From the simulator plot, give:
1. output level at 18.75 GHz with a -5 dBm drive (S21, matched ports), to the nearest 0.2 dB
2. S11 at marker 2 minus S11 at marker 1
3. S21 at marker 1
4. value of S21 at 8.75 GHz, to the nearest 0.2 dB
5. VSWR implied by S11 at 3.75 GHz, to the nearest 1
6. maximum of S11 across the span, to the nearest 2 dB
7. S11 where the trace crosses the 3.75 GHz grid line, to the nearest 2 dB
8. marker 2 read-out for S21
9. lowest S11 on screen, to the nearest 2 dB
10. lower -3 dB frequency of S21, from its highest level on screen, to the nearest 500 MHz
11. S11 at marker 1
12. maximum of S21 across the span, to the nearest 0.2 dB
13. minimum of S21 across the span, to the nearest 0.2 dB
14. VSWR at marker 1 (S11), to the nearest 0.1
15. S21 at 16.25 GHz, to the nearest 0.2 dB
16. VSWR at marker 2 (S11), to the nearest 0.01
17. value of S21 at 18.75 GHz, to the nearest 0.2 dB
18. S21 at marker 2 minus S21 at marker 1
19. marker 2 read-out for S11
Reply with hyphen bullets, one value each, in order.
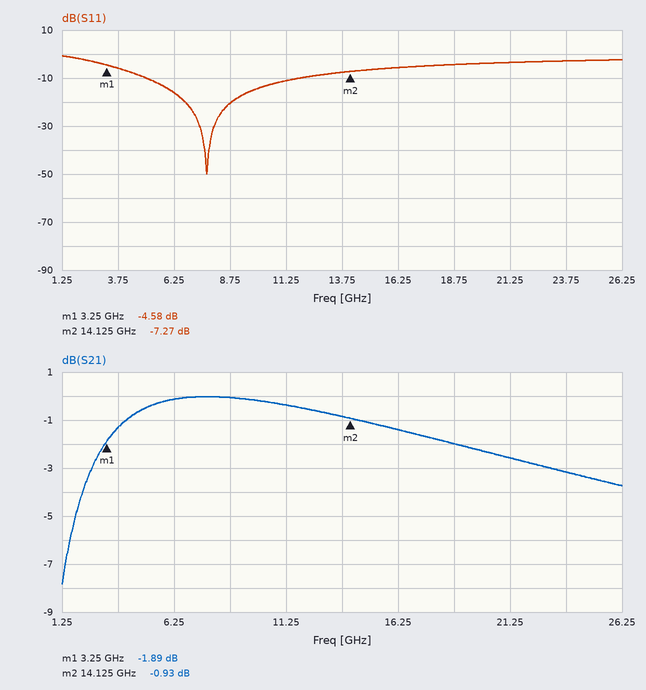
- -7.0 dBm
- -2.69 dB
- -1.89 dB
- 0.0 dB
- 3
- 0 dB
- -6 dB
- -0.93 dB
- -50 dB
- 2.5 GHz
- -4.58 dB
- 0.0 dB
- -7.8 dB
- 3.9
- -1.4 dB
- 2.53
- -2.0 dB
- 0.96 dB
- -7.27 dB
